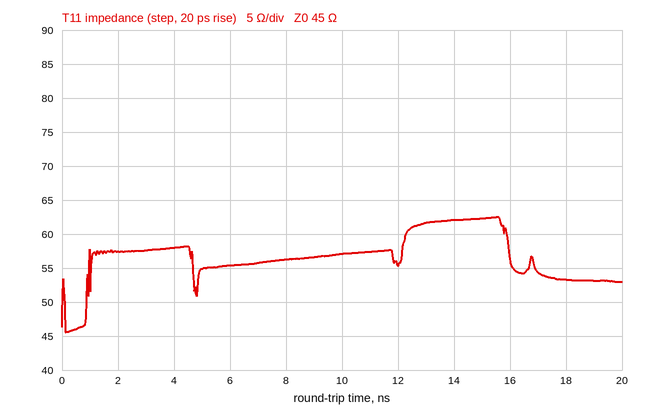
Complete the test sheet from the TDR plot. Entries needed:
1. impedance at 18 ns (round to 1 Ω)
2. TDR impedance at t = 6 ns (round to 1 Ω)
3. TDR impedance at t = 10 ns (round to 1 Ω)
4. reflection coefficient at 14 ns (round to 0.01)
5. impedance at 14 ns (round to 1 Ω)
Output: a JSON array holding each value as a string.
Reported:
["53 Ω", "55 Ω", "57 Ω", "+0.16", "62 Ω"]
